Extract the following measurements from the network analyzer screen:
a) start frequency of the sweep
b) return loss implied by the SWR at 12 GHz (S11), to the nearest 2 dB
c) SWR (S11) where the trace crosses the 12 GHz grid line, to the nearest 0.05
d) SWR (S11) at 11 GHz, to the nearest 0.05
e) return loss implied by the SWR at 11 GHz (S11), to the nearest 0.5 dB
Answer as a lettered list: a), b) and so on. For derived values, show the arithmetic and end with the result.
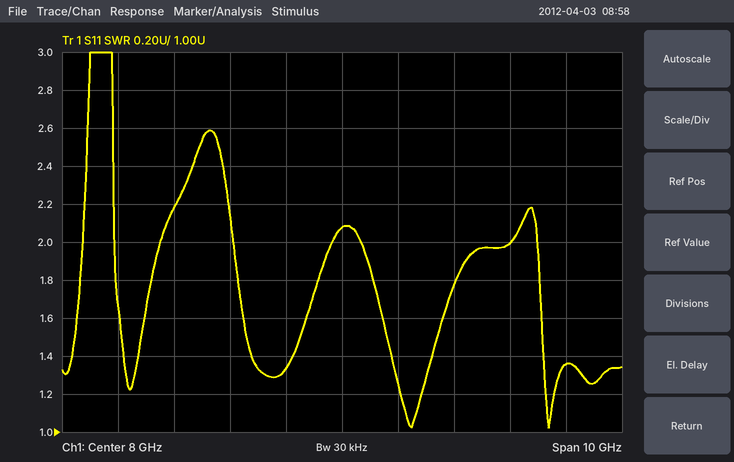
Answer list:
a) 3 GHz
b) −20 log10((1.35 − 1)/(1.35 + 1)) ≈ 16 dB
c) 1.35
d) 2.00
e) −20 log10((2 − 1)/(2 + 1)) ≈ 9.5 dB
